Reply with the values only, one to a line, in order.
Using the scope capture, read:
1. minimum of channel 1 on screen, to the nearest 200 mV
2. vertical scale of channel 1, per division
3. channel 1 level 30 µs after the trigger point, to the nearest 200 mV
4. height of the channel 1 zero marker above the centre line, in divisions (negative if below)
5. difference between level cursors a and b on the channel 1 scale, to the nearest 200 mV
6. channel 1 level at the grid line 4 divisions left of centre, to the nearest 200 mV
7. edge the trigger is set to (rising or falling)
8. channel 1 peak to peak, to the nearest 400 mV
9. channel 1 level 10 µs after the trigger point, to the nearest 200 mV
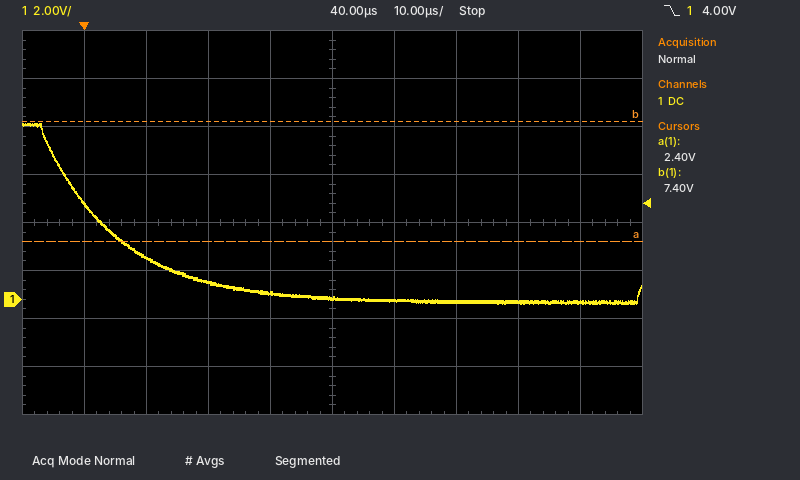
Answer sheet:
-200 mV
2 V
200 mV
-1.6 div
5.0 V
4.0 V
falling
7.6 V
1.8 V
